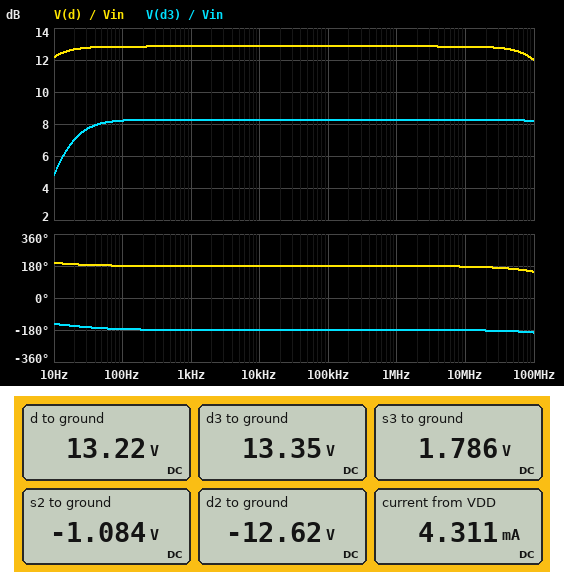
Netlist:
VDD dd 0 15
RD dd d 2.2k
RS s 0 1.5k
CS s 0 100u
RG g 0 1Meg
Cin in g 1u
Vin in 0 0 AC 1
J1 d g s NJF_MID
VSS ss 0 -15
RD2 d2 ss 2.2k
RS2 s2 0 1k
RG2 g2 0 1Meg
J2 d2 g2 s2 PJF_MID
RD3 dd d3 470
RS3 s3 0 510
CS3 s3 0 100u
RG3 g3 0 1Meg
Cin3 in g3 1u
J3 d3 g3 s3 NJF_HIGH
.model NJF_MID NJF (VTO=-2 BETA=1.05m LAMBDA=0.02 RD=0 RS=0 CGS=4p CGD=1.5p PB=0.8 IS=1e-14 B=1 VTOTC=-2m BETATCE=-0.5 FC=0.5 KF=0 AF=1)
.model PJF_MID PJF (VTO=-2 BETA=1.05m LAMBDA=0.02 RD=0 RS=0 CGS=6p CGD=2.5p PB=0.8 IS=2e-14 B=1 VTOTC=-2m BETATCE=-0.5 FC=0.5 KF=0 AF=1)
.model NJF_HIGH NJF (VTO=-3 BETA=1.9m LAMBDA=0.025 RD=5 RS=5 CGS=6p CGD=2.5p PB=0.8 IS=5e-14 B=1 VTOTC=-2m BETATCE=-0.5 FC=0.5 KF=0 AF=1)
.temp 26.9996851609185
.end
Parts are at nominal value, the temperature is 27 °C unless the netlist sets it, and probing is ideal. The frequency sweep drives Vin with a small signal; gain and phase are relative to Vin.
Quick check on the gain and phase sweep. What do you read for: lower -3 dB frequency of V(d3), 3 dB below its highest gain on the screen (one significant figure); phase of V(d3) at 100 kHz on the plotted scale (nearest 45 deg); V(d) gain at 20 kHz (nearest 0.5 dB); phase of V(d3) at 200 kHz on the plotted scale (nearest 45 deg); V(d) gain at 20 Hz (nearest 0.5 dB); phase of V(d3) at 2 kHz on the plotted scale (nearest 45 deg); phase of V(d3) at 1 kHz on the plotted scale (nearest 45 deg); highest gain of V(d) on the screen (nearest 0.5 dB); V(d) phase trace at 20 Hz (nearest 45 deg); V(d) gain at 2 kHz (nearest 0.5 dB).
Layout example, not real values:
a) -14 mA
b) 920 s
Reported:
a) 10 Hz
b) -180 deg
c) 13.0 dB
d) -180 deg
e) 12.5 dB
f) -180 deg
g) -180 deg
h) 13.0 dB
i) 180 deg
j) 13.0 dB
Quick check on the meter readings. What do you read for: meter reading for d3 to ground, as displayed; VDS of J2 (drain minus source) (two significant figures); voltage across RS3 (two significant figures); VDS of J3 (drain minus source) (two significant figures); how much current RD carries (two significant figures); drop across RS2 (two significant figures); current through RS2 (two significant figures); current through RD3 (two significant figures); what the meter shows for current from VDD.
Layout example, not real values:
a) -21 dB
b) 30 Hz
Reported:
a) 13.35 V
b) -12 V
c) 1.8 V
d) 12 V
e) 810 µA
f) 1.1 V
g) 1.1 mA
h) 3.5 mA
i) 4.311 mA
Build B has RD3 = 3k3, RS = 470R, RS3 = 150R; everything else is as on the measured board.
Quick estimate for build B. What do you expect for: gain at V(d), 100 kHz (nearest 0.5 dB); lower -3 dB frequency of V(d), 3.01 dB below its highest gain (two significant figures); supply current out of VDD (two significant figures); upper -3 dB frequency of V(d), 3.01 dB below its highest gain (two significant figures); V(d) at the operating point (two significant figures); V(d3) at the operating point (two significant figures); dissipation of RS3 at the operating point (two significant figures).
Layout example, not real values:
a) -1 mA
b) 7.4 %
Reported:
a) 16.0 dB
b) 6.3 Hz
c) 5.9 mA
d) 200 MHz
e) 11 V
f) 1.2 V
g) 2.6 mW
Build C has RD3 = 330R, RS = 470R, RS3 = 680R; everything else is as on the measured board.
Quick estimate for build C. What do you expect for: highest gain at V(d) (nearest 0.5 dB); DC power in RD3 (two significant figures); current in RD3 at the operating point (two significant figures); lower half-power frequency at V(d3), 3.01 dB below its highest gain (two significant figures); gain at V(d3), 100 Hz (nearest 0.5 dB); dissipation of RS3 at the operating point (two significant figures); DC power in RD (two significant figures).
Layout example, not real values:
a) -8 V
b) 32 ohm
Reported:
a) 16.0 dB
b) 2.6 mW
c) 2.8 mA
d) 9.9 Hz
e) 4.5 dB
f) 5.4 mW
g) 6.8 mW
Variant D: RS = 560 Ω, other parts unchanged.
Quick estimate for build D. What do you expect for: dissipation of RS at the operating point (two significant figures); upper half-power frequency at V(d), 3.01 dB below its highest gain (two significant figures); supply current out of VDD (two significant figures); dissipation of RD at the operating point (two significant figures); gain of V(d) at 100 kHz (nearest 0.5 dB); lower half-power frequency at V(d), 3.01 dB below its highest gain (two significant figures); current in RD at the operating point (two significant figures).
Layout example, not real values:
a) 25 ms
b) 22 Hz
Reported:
a) 1.4 mW
b) 210 MHz
c) 5.1 mA
d) 5.5 mW
e) 15.5 dB
f) 5.9 Hz
g) 1.6 mA
